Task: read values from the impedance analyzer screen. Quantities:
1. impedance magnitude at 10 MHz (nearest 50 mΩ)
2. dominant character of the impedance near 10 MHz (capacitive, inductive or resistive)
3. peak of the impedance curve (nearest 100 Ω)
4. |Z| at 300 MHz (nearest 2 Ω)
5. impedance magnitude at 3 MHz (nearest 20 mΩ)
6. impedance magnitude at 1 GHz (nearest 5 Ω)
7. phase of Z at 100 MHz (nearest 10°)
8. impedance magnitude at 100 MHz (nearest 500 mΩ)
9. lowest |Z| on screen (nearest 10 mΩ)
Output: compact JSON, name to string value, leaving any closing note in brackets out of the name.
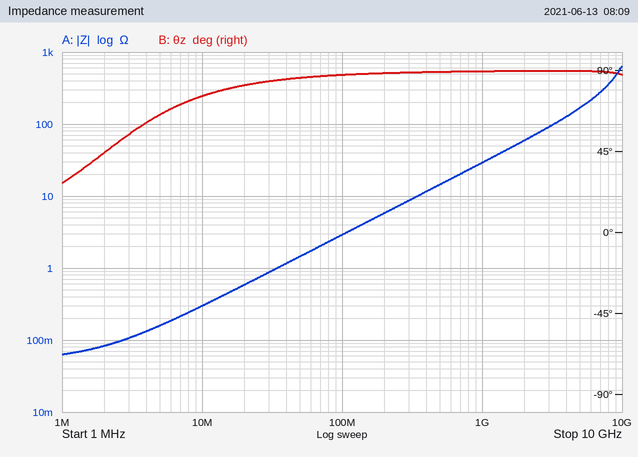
{"impedance magnitude at 10 MHz": "300 mΩ", "dominant character of the impedance near 10 MHz": "inductive", "peak of the impedance curve": "600 Ω", "|Z| at 300 MHz": "8 Ω", "impedance magnitude at 3 MHz": "100 mΩ", "impedance magnitude at 1 GHz": "30 Ω", "phase of Z at 100 MHz": "90°", "impedance magnitude at 100 MHz": "3.0 Ω", "lowest |Z| on screen": "60 mΩ"}
